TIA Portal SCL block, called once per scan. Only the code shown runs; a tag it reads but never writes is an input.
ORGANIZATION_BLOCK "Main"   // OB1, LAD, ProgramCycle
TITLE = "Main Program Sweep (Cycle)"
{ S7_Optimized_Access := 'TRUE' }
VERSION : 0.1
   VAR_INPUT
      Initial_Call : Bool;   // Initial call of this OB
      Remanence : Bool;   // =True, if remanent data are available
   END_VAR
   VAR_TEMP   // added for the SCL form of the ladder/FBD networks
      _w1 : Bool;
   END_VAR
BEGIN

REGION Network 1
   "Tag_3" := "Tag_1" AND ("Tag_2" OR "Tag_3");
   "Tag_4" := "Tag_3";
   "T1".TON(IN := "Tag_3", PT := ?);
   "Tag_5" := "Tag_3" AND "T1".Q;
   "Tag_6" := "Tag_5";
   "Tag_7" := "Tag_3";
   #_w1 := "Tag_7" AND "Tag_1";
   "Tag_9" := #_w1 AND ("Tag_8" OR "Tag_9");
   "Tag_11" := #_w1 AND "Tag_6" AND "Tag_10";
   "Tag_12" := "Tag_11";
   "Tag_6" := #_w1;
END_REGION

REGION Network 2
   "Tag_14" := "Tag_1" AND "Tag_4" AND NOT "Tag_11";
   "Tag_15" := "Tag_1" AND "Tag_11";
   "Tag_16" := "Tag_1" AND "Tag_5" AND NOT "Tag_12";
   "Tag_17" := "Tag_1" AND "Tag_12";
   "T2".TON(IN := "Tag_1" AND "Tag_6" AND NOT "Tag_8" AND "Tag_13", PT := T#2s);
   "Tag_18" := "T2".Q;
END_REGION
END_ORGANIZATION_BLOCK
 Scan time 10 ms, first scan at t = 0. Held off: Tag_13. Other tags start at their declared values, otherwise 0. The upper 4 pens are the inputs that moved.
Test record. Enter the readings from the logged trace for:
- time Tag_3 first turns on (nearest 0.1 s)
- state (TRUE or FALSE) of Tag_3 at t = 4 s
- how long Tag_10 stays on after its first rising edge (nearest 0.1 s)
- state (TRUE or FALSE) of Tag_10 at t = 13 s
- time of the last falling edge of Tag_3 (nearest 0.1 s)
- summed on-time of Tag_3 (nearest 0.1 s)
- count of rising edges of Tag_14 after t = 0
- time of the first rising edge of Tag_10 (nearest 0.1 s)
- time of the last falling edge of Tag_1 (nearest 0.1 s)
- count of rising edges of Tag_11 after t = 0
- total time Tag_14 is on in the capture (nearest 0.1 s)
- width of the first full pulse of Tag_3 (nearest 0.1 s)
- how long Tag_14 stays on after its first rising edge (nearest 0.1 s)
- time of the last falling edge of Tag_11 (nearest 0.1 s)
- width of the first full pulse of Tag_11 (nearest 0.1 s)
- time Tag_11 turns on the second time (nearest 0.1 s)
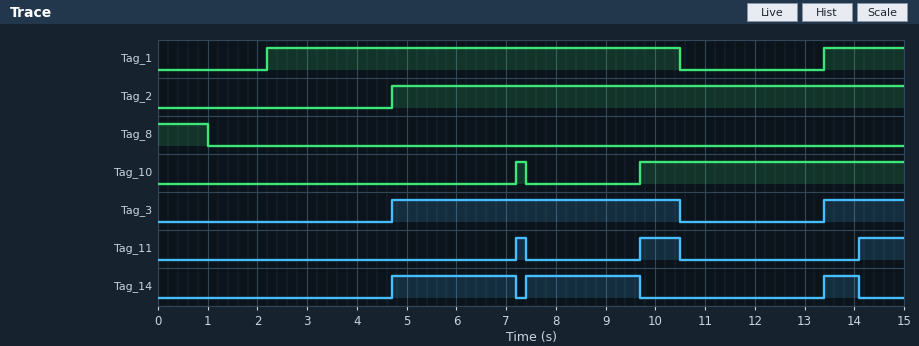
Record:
4.7 s
FALSE
0.2 s
TRUE
10.5 s
7.4 s
3
7.2 s
10.5 s
3
5.5 s
5.8 s
2.5 s
10.5 s
0.2 s
9.7 s
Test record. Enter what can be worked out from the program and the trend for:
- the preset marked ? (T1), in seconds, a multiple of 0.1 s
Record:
0.7 s
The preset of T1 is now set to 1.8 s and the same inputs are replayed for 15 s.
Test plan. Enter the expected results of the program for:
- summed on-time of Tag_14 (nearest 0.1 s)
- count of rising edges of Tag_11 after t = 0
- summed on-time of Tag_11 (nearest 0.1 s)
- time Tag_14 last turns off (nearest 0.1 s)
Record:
6.4 s
2
1.0 s
9.7 s
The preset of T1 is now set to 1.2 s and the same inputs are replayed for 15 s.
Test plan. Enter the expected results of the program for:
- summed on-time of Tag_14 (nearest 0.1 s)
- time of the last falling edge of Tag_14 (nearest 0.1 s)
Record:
6.0 s
14.6 s
